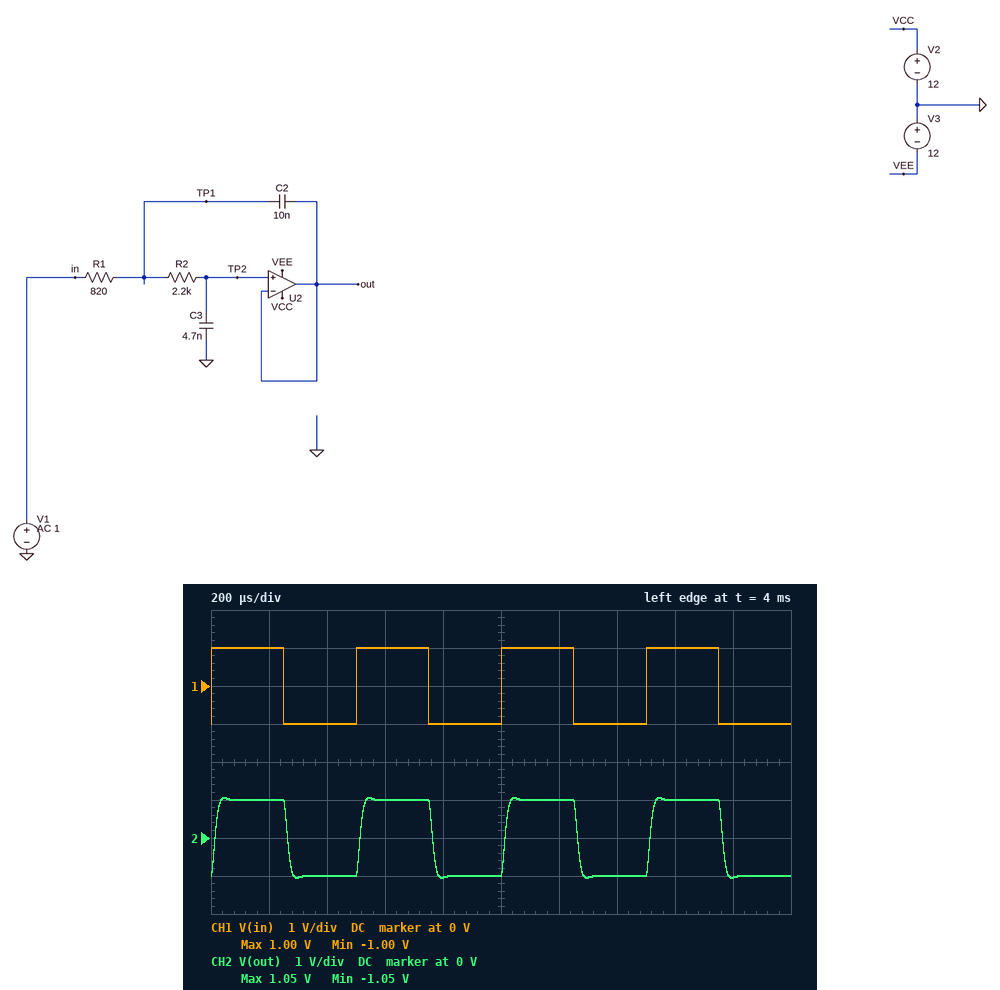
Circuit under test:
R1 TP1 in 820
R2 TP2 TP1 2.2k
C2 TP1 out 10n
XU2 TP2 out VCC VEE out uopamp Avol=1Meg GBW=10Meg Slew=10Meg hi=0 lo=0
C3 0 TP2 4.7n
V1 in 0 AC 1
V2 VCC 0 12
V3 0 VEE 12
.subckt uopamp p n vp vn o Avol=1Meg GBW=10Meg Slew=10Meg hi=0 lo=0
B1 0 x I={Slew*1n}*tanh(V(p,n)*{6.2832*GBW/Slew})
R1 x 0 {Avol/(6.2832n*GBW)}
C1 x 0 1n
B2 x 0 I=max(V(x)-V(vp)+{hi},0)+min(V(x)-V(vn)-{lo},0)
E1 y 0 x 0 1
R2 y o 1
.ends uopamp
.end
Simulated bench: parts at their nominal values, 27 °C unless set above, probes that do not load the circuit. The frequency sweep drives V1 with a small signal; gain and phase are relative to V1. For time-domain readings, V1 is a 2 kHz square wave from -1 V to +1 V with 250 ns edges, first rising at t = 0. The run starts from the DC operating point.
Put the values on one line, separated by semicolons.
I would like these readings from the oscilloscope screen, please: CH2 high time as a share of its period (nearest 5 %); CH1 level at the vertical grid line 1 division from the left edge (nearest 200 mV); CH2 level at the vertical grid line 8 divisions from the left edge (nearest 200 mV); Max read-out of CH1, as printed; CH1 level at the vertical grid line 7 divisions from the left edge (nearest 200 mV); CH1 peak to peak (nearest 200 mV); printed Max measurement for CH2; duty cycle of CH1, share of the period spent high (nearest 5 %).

50 %; 1.0 V; 1.0 V; 1.00 V; -1.0 V; 2.0 V; 1.05 V; 50 %
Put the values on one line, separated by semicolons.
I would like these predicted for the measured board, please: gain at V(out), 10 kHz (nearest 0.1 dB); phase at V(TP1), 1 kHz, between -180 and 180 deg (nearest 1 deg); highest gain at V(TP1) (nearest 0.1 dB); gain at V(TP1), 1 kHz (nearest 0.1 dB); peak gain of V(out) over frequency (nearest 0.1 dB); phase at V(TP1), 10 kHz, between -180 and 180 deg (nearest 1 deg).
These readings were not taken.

-0.9 dB; -1 deg; 0.6 dB; 0 dB; 0 dB; -20 deg
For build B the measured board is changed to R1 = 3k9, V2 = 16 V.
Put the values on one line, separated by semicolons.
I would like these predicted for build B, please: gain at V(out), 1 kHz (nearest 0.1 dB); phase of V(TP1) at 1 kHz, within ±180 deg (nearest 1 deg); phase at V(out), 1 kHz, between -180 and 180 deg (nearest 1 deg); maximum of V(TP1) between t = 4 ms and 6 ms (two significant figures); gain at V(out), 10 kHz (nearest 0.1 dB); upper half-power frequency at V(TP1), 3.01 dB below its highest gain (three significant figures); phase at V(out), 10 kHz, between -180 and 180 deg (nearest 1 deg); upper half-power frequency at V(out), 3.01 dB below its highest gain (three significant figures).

0 dB; -7 deg; -10 deg; 1.1 V; -5.6 dB; 8.89 kHz; -108 deg; 7.85 kHz
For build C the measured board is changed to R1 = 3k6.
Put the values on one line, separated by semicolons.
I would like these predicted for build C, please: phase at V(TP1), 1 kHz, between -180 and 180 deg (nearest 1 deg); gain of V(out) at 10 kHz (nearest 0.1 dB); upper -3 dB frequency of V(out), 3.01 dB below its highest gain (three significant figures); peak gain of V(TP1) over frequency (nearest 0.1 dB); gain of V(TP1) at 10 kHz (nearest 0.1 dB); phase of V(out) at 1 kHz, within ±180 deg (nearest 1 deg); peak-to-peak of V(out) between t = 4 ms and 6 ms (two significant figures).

-6 deg; -5.0 dB; 8.26 kHz; 0.1 dB; -3.5 dB; -10 deg; 2.2 V
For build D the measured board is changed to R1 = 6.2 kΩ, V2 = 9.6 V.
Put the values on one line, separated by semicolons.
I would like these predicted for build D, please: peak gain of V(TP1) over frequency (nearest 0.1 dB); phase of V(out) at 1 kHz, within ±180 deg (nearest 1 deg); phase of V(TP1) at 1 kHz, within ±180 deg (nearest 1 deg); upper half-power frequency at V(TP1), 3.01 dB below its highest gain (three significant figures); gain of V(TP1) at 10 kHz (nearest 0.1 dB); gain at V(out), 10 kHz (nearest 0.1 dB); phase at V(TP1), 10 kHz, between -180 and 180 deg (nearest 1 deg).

0 dB; -14 deg; -11 deg; 6.13 kHz; -7.8 dB; -9.3 dB; -89 deg
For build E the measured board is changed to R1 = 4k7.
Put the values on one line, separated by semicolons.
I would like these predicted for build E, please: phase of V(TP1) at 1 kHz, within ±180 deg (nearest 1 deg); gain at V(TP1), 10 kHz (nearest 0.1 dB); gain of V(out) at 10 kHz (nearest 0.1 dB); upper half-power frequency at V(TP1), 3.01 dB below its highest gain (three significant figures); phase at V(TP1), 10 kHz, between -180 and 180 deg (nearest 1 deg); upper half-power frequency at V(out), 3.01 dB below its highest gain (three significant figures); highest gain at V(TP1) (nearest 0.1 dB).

-8 deg; -5.5 dB; -7.0 dB; 7.73 kHz; -81 deg; 6.93 kHz; 0 dB
